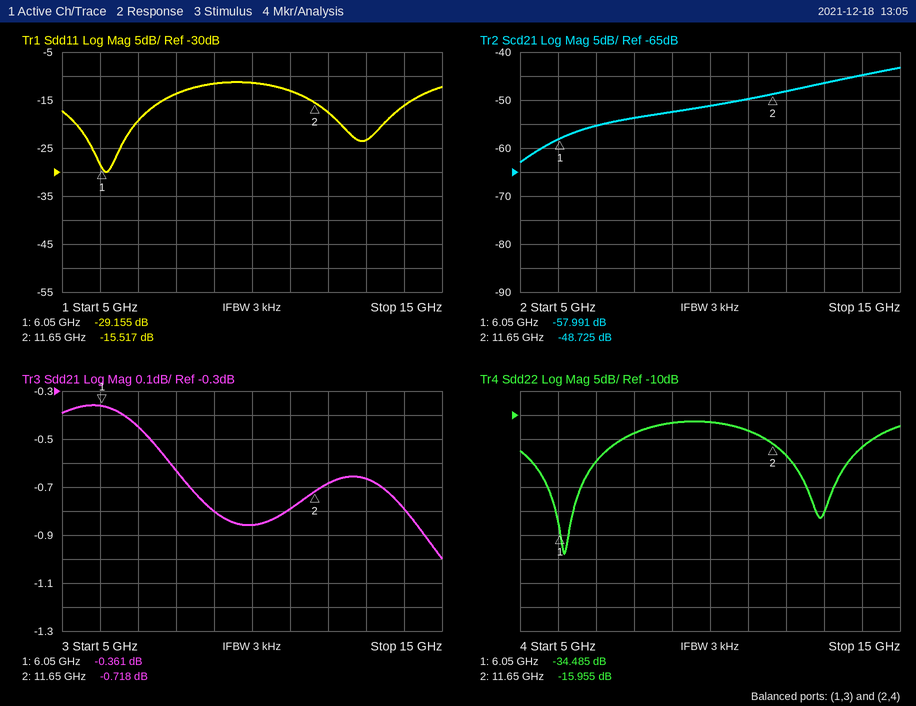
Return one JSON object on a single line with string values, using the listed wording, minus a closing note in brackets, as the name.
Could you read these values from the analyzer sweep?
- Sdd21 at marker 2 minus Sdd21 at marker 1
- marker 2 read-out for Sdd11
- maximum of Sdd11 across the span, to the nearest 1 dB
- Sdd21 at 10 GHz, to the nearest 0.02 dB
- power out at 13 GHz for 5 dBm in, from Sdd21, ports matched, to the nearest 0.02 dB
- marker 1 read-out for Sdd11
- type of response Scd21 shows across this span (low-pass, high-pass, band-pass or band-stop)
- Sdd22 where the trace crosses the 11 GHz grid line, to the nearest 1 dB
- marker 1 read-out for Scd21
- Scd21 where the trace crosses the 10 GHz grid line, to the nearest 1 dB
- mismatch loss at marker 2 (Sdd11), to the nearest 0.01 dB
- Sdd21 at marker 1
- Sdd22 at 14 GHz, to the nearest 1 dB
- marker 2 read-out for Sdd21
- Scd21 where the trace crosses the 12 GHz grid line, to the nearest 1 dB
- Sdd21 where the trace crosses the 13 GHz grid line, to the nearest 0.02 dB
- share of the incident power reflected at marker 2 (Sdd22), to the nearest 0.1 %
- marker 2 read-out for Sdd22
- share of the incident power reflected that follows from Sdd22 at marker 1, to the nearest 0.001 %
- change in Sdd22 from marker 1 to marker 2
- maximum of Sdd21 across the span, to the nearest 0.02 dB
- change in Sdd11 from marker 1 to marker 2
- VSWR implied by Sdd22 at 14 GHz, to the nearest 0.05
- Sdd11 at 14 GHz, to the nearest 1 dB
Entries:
{"Sdd21 at marker 2 minus Sdd21 at marker 1": "-0.357 dB", "marker 2 read-out for Sdd11": "-15.517 dB", "maximum of Sdd11 across the span, to the nearest 1 dB": "-11 dB", "Sdd21 at 10 GHz, to the nearest 0.02 dB": "-0.86 dB", "power out at 13 GHz for 5 dBm in, from Sdd21, ports matched, to the nearest 0.02 dB": "4.34 dBm", "marker 1 read-out for Sdd11": "-29.155 dB", "type of response Scd21 shows across this span": "high-pass", "Sdd22 where the trace crosses the 11 GHz grid line, to the nearest 1 dB": "-13 dB", "marker 1 read-out for Scd21": "-57.991 dB", "Scd21 where the trace crosses the 10 GHz grid line, to the nearest 1 dB": "-51 dB", "mismatch loss at marker 2 (Sdd11), to the nearest 0.01 dB": "0.12 dB", "Sdd21 at marker 1": "-0.361 dB", "Sdd22 at 14 GHz, to the nearest 1 dB": "-17 dB", "marker 2 read-out for Sdd21": "-0.718 dB", "Scd21 where the trace crosses the 12 GHz grid line, to the nearest 1 dB": "-48 dB", "Sdd21 where the trace crosses the 13 GHz grid line, to the nearest 0.02 dB": "-0.66 dB", "share of the incident power reflected at marker 2 (Sdd22), to the nearest 0.1 %": "2.5 %", "marker 2 read-out for Sdd22": "-15.955 dB", "share of the incident power reflected that follows from Sdd22 at marker 1, to the nearest 0.001 %": "0.036 %", "change in Sdd22 from marker 1 to marker 2": "18.530 dB", "maximum of Sdd21 across the span, to the nearest 0.02 dB": "-0.36 dB", "change in Sdd11 from marker 1 to marker 2": "13.638 dB", "VSWR implied by Sdd22 at 14 GHz, to the nearest 0.05": "1.35", "Sdd11 at 14 GHz, to the nearest 1 dB": "-16 dB"}
